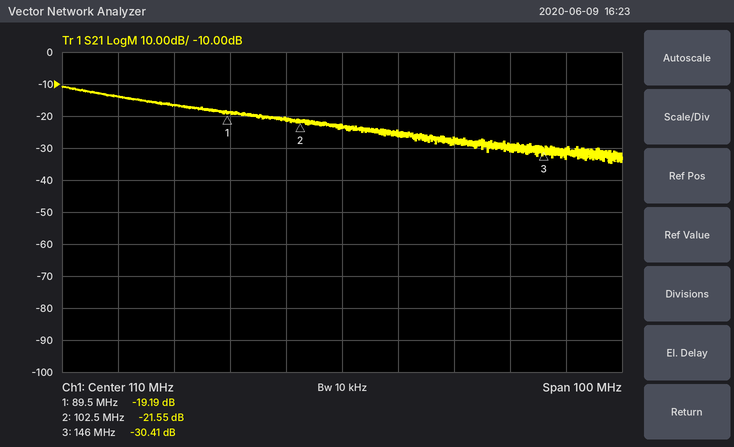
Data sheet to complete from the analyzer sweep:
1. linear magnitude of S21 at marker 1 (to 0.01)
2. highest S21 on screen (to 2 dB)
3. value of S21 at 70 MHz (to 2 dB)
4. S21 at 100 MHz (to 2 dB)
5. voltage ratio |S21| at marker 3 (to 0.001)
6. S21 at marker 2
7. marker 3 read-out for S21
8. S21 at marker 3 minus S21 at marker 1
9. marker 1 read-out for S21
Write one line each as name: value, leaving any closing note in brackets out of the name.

linear magnitude of S21 at marker 1: 0.11
highest S21 on screen: -10 dB
value of S21 at 70 MHz: -14 dB
S21 at 100 MHz: -22 dB
voltage ratio |S21| at marker 3: 0.030
S21 at marker 2: -21.55 dB
marker 3 read-out for S21: -30.41 dB
S21 at marker 3 minus S21 at marker 1: -11.22 dB
marker 1 read-out for S21: -19.19 dB
